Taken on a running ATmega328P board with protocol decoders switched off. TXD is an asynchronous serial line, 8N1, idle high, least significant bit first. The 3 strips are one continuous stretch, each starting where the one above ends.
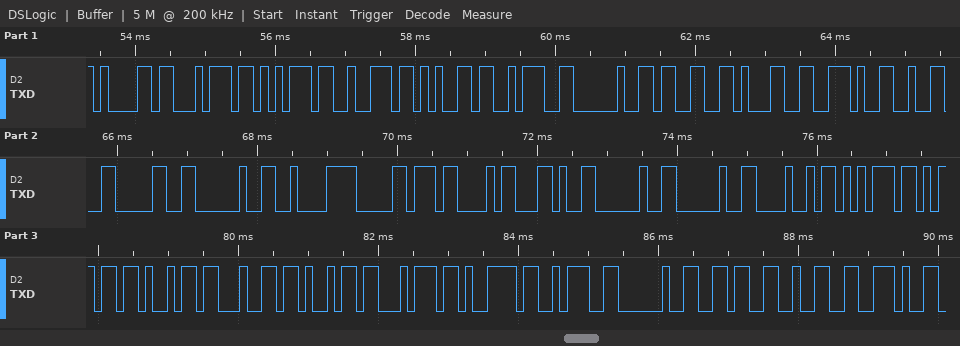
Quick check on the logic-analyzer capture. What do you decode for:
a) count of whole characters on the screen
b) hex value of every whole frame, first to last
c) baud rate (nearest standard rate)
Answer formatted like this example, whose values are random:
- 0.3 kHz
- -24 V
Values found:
- 32
- 61 74 75 72 65 3A 20 33 31 2E 32 30 20 C2 B0 43 2C 20 20 48 75 6D 69 64 69 74 79 3A 20 36 32 2E
- 9600 baud
